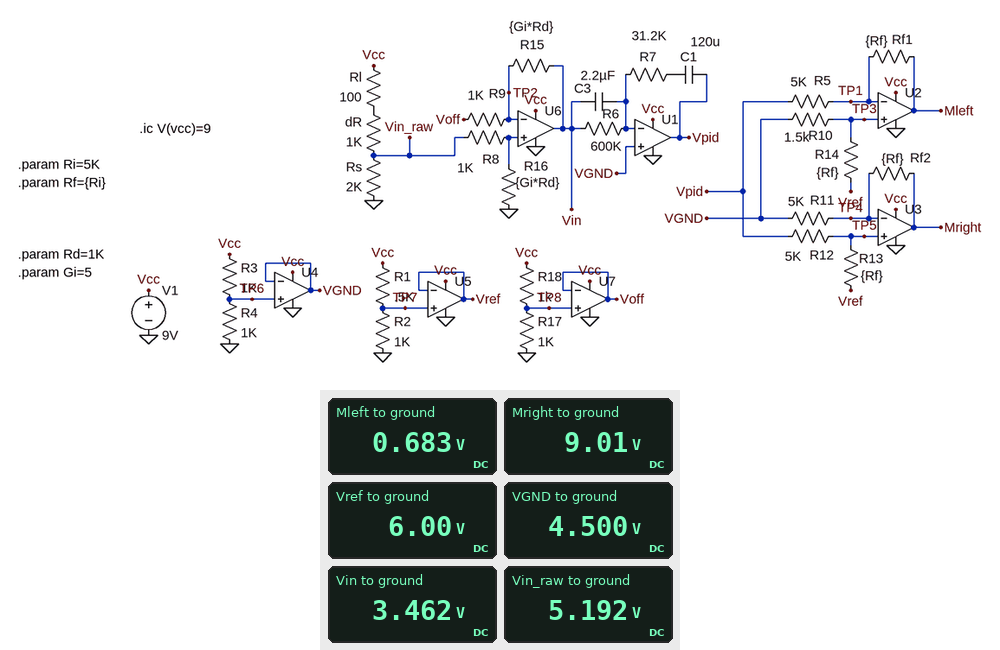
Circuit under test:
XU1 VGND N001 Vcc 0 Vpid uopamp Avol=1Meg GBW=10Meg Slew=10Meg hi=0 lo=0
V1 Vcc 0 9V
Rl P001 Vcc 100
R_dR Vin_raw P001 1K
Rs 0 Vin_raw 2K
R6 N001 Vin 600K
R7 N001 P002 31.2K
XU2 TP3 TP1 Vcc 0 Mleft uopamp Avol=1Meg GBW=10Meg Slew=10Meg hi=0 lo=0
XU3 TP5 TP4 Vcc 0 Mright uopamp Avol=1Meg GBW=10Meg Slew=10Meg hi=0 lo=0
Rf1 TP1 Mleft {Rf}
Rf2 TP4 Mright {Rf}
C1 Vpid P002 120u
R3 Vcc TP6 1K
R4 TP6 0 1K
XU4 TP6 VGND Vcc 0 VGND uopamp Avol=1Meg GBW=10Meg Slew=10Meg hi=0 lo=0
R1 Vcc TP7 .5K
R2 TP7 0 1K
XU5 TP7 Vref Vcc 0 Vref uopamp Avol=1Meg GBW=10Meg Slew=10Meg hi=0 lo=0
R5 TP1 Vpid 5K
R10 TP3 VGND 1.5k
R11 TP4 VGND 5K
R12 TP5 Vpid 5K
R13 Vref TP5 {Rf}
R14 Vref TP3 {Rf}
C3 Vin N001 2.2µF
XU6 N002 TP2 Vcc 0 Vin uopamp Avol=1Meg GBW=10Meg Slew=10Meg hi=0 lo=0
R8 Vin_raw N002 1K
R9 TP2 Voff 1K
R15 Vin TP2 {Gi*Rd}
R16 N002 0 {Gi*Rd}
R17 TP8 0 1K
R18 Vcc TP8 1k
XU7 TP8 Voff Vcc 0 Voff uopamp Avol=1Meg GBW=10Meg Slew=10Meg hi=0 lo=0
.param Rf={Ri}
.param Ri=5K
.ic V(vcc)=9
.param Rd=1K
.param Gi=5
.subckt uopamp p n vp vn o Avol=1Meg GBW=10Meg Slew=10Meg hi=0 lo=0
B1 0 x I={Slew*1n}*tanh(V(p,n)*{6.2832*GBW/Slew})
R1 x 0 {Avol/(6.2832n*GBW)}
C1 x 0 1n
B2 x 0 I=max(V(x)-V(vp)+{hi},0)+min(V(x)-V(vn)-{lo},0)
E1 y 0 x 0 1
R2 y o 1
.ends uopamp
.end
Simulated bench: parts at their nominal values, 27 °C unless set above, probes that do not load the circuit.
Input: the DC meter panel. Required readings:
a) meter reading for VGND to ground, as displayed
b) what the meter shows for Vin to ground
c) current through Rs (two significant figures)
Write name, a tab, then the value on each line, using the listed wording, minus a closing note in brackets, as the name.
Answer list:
meter reading for VGND to ground, as displayed	4.500 V
what the meter shows for Vin to ground	3.462 V
current through Rs	2.6 mA
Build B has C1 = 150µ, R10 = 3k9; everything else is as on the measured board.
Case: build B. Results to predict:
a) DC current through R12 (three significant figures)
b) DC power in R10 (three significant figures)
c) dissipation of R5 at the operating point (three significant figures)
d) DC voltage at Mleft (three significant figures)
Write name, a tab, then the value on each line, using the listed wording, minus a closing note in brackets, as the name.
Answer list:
DC current through R12	301 µA
DC power in R10	111 µW
dissipation of R5 at the operating point	2.97 mW
DC voltage at Mleft	1.31 V
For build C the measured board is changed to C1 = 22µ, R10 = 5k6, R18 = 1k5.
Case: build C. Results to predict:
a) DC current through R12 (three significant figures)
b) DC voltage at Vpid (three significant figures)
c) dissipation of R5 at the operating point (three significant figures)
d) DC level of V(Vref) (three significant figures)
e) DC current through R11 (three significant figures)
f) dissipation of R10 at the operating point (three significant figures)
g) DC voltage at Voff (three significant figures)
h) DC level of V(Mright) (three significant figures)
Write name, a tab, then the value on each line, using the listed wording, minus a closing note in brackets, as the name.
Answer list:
DC current through R12	601 µA
DC voltage at Vpid	-8.24 mV
dissipation of R5 at the operating point	4.07 mW
DC level of V(Vref)	6.00 V
DC current through R11	301 µA
dissipation of R10 at the operating point	112 µW
DC voltage at Voff	3.60 V
DC level of V(Mright)	1.49 V
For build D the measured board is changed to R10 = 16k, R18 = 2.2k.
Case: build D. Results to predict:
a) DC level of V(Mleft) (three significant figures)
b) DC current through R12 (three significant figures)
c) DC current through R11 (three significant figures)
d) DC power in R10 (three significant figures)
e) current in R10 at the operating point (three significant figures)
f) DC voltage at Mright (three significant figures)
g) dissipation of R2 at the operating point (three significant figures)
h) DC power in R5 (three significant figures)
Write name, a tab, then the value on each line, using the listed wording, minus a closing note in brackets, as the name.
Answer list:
DC level of V(Mleft)	9.01 V
DC current through R12	601 µA
DC current through R11	301 µA
DC power in R10	81.6 µW
current in R10 at the operating point	71.4 µA
DC voltage at Mright	1.49 V
dissipation of R2 at the operating point	36.0 mW
DC power in R5	4.07 mW
